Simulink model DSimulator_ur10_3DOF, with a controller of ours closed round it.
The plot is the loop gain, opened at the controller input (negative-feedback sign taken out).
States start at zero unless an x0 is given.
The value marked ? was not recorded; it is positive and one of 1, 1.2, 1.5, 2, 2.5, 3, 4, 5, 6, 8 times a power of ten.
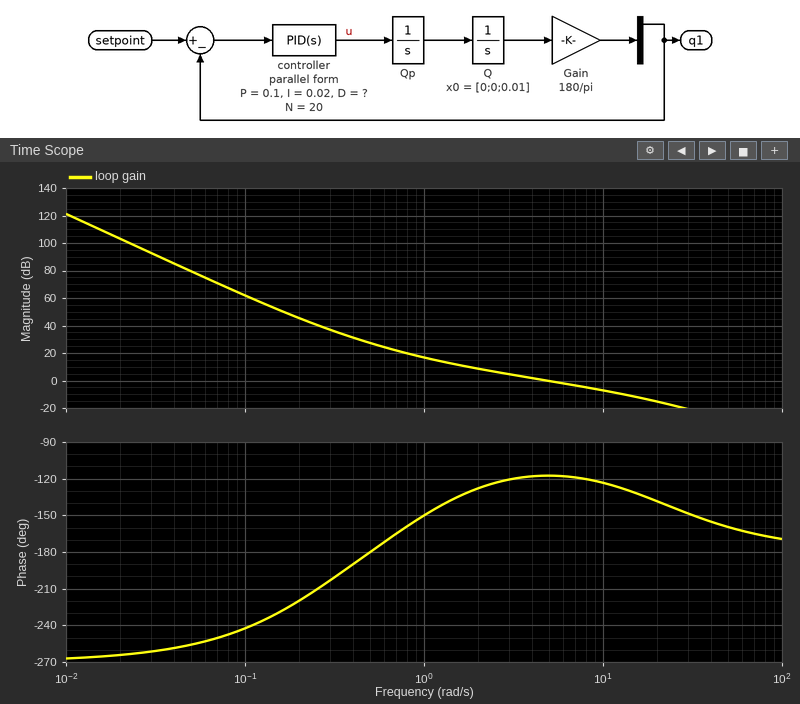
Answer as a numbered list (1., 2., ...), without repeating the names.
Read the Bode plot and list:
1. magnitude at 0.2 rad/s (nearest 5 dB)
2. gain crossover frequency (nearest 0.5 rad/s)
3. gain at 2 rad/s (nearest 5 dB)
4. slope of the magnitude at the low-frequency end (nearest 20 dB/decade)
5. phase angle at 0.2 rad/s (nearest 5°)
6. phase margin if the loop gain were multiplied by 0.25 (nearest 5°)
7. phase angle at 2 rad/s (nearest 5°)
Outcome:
1. 45 dB
2. 5.0 rad/s
3. 10 dB
4. -60 dB/decade
5. -220°
6. 45°
7. -130°
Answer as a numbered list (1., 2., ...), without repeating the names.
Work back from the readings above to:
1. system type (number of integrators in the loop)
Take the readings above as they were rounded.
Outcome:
1. 3
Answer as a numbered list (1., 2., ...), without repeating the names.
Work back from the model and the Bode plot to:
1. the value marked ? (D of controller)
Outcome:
1. 0.08
